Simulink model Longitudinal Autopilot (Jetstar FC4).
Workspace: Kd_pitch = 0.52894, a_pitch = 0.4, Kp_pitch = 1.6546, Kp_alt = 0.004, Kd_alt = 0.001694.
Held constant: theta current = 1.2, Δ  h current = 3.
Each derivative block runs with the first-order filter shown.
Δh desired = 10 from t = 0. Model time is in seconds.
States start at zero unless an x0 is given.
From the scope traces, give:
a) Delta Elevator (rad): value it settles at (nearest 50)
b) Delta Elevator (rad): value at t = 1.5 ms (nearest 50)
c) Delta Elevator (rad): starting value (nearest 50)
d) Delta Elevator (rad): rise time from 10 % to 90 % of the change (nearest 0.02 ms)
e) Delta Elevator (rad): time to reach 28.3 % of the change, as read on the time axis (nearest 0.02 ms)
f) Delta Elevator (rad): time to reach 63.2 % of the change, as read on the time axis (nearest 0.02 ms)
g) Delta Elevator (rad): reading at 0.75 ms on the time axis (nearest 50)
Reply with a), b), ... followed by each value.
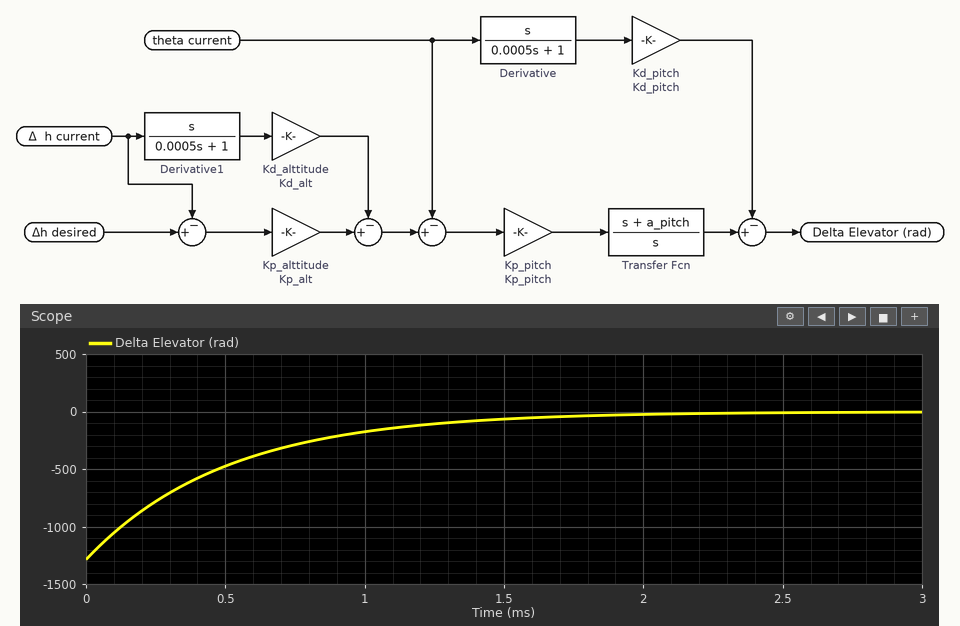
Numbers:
a) 0
b) -50
c) -1300
d) 1.10 ms
e) 0.16 ms
f) 0.50 ms
g) -300
